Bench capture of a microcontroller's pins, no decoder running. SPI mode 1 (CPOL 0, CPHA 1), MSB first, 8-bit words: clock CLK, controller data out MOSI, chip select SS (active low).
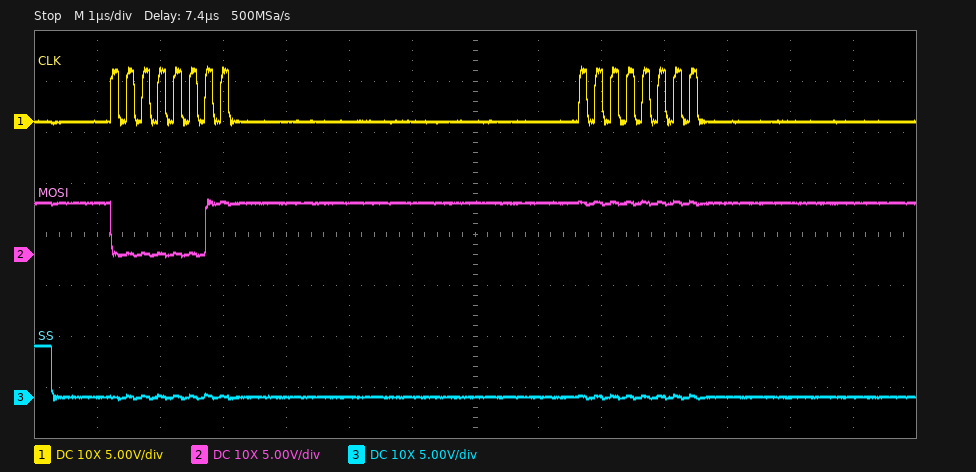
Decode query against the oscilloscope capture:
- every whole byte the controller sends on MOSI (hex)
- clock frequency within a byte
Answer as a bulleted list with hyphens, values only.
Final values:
- 03 FF
- 4 MHz
